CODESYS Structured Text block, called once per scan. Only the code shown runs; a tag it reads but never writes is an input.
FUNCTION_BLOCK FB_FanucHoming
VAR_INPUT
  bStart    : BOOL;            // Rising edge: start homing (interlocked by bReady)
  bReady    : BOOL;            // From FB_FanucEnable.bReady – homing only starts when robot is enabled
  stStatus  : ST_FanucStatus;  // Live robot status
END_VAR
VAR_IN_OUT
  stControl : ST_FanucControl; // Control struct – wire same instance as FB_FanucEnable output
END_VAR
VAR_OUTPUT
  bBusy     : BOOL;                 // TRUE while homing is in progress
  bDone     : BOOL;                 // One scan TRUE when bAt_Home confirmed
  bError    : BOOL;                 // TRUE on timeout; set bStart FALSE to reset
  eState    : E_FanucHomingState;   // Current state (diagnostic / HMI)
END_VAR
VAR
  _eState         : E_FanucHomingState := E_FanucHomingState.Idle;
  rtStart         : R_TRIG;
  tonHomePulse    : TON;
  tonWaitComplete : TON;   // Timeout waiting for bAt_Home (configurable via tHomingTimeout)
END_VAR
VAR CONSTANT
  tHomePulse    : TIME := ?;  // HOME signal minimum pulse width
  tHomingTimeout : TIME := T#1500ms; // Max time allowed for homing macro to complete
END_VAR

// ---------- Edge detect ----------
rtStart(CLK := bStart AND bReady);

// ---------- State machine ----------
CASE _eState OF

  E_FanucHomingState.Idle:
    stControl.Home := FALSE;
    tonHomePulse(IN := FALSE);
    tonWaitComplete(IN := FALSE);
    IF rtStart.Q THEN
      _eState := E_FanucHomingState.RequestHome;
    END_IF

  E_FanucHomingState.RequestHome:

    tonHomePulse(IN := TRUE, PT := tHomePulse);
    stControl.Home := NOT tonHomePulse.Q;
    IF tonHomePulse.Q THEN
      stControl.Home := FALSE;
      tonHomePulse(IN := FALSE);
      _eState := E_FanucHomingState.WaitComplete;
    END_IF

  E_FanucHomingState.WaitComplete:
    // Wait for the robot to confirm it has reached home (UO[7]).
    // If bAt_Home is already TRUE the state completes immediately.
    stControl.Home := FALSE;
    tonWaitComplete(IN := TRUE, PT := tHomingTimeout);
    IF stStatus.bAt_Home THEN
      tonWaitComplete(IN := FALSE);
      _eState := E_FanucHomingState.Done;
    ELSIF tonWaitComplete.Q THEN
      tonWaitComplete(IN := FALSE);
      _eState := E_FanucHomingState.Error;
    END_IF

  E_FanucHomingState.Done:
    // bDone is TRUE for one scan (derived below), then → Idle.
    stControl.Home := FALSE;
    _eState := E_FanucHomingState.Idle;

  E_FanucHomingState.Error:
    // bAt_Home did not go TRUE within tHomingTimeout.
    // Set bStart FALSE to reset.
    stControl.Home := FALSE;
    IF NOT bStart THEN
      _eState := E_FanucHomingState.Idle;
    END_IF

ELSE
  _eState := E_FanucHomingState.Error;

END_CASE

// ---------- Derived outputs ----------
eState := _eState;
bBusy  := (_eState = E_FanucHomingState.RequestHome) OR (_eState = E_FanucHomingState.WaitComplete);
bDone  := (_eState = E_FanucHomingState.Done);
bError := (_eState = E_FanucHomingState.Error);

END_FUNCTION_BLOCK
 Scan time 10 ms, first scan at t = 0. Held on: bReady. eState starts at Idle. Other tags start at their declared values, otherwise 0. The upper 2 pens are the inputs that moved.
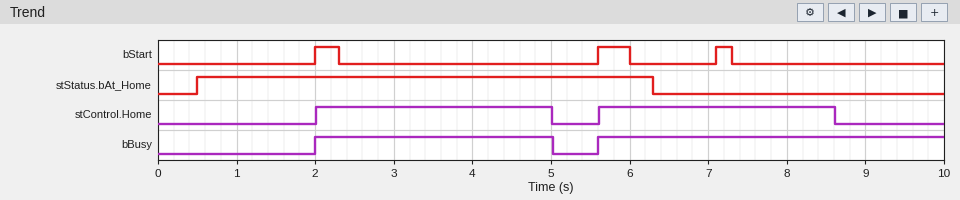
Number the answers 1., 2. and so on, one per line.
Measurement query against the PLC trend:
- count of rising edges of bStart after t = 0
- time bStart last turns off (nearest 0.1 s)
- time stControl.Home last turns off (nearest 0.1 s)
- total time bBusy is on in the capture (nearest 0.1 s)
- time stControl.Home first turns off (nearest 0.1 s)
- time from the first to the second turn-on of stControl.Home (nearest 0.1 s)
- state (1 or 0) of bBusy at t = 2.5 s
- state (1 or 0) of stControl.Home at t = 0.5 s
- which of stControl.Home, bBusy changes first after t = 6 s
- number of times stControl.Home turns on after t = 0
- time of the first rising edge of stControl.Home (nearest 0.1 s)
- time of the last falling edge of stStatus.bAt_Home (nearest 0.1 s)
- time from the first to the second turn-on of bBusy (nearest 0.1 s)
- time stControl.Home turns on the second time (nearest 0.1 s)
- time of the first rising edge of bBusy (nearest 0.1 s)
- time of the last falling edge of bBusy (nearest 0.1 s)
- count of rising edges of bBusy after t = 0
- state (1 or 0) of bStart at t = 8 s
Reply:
1. 3
2. 7.3 s
3. 8.6 s
4. 7.4 s
5. 5.0 s
6. 3.6 s
7. 1
8. 0
9. stControl.Home
10. 2
11. 2.0 s
12. 6.3 s
13. 3.6 s
14. 5.6 s
15. 2.0 s
16. 5.0 s
17. 2
18. 0
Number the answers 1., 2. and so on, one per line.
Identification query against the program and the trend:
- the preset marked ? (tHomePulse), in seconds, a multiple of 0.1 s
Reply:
1. 3.0 s
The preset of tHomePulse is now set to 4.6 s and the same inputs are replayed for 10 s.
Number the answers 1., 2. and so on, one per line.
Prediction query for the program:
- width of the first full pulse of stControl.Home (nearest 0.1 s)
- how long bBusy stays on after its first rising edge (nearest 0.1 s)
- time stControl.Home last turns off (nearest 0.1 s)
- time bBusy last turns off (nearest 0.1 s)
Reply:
1. 4.6 s
2. 6.1 s
3. 6.6 s
4. 8.1 s
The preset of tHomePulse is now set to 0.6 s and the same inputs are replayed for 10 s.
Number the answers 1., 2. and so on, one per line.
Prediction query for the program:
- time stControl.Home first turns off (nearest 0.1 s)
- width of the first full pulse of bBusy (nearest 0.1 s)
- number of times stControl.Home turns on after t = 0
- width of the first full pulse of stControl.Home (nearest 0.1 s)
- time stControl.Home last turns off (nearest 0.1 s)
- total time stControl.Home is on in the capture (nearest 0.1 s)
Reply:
1. 2.6 s
2. 0.6 s
3. 3
4. 0.6 s
5. 7.7 s
6. 1.8 s
